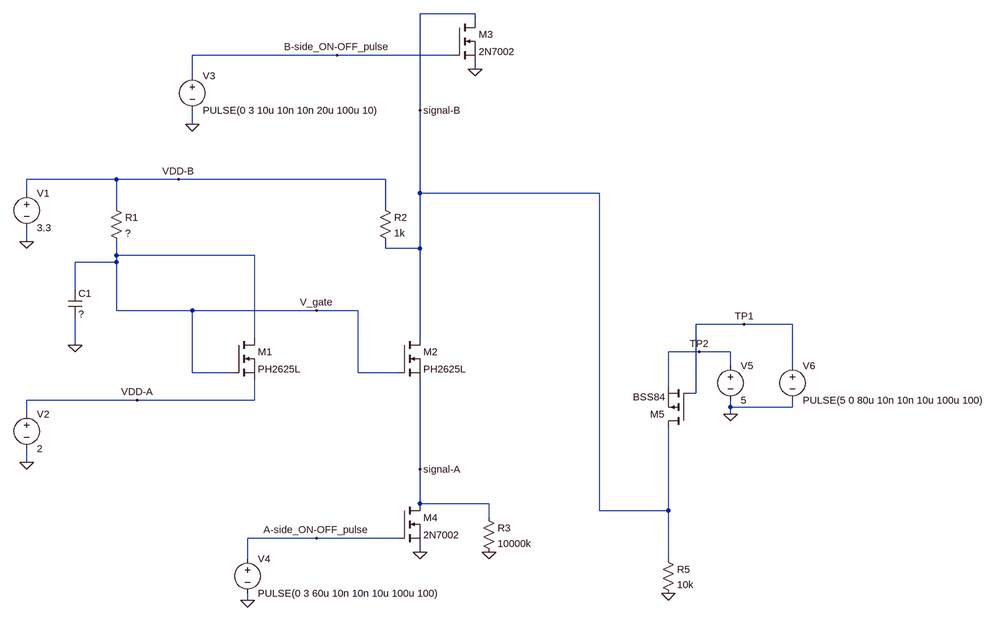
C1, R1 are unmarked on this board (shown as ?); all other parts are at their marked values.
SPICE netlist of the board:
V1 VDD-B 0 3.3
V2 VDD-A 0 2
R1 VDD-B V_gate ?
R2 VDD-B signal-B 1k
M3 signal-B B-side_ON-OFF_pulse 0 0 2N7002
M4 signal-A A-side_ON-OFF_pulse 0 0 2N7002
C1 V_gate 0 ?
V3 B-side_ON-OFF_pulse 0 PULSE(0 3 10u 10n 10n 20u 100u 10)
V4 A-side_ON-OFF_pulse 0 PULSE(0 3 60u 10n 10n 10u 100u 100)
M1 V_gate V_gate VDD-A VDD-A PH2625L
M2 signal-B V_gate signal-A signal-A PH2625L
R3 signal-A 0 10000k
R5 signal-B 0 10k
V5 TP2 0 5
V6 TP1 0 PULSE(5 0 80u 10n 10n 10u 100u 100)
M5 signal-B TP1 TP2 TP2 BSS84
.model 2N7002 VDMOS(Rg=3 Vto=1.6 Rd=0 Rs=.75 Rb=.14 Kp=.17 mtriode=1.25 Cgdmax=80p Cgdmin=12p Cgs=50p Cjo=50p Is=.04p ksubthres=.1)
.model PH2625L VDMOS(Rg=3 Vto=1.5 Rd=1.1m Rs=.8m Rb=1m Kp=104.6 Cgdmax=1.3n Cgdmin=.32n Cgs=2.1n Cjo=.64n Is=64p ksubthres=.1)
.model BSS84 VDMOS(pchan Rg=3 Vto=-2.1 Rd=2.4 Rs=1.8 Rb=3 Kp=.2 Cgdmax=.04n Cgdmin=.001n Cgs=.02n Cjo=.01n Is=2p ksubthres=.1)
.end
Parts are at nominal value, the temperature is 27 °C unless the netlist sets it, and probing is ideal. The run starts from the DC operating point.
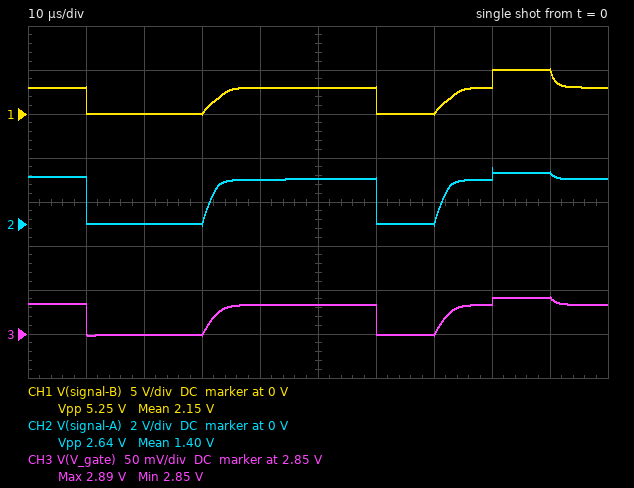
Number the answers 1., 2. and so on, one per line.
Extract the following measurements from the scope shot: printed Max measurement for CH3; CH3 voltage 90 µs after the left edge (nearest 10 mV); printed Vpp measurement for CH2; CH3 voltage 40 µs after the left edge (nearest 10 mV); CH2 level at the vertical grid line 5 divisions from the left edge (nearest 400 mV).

1. 2.89 V
2. 2.89 V
3. 2.64 V
4. 2.88 V
5. 2.0 V
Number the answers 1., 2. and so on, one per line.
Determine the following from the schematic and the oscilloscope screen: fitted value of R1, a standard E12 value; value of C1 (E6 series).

1. 180 kΩ
2. 220 nF
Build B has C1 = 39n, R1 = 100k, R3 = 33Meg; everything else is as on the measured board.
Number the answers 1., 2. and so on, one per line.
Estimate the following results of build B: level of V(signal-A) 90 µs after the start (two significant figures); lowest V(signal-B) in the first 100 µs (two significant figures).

1. 2.4 V
2. -79 mV
